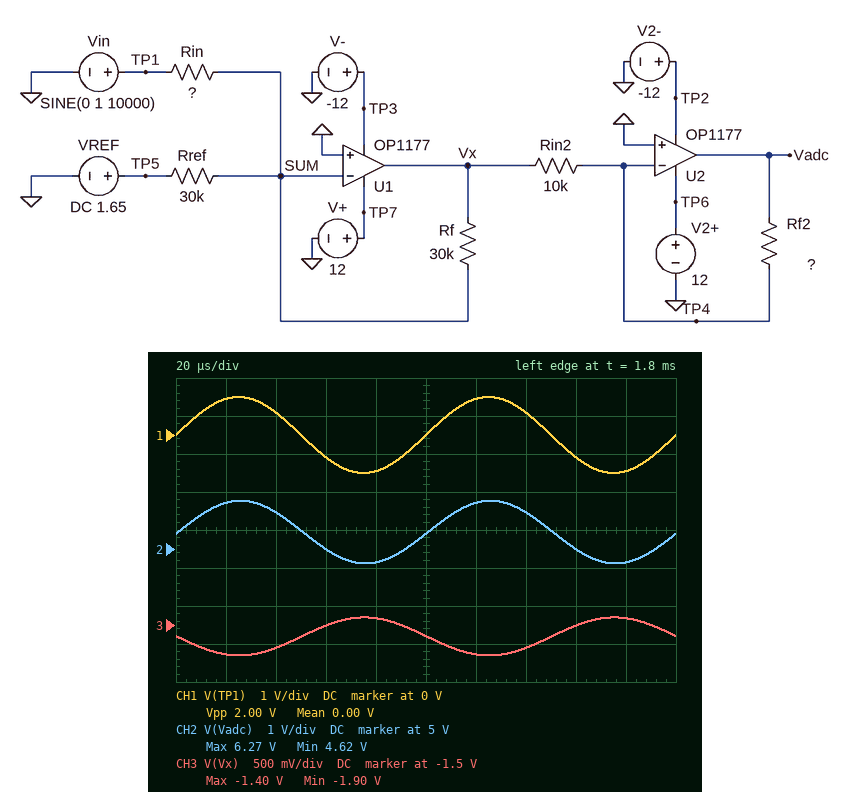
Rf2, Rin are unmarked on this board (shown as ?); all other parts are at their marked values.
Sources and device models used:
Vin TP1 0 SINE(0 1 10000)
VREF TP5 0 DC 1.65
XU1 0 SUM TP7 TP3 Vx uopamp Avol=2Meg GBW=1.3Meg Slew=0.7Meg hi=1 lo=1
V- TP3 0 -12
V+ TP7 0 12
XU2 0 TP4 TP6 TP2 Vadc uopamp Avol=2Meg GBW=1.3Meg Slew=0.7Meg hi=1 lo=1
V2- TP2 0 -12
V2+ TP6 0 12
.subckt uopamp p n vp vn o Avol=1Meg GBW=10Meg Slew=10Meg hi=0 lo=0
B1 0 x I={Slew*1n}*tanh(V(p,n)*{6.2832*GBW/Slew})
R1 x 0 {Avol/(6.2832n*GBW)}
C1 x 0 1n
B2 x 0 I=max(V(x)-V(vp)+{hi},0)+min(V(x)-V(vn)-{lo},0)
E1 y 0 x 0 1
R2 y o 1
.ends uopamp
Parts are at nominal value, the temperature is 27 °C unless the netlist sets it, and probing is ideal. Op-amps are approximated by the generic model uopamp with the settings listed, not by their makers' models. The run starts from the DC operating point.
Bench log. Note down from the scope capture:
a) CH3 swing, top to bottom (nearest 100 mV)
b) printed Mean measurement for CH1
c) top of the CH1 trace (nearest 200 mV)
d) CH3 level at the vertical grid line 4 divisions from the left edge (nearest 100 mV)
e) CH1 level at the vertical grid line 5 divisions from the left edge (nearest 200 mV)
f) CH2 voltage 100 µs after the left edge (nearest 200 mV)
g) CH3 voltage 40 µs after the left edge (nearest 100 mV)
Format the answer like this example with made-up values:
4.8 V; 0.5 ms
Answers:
500 mV; 0.00 V; 1.0 V; -1.4 V; 0 V; 5.4 V; -1.8 V
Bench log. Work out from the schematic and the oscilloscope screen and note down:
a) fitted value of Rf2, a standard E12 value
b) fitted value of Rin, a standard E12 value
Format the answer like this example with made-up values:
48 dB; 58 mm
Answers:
33 kΩ; 120 kΩ
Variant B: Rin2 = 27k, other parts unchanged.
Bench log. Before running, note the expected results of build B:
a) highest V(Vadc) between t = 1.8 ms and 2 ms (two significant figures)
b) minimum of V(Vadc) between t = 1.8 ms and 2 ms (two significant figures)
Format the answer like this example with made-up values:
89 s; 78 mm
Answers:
2.3 V; 1.7 V
